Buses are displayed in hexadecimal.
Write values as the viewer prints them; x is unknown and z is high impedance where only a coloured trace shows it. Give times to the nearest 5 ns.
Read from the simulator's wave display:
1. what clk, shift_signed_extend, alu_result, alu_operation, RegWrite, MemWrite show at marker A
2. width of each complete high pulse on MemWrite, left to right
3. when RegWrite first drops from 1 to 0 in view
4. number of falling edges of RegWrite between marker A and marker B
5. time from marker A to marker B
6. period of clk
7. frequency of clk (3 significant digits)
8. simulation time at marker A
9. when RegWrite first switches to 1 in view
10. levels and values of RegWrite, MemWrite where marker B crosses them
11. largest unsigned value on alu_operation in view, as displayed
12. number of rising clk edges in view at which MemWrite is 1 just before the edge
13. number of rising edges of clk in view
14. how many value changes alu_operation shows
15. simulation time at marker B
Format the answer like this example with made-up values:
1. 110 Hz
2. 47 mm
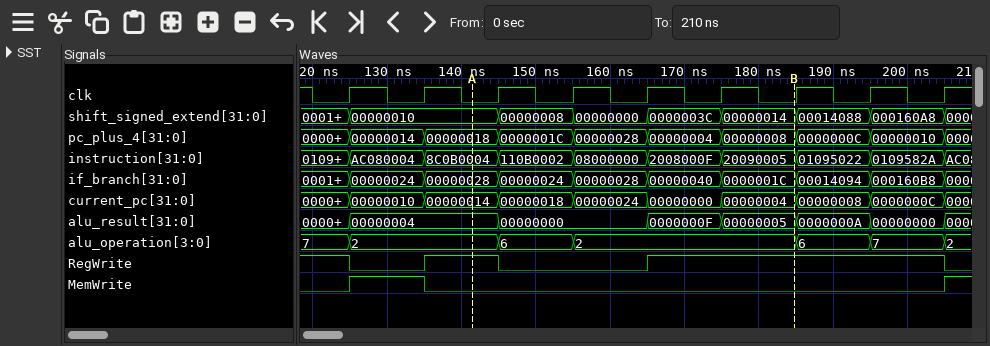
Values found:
1. clk=0, shift_signed_extend=00000010, alu_result=00000004, alu_operation=2, RegWrite=1, MemWrite=0
2. 10 ns
3. 125 ns
4. 1
5. 45 ns
6. 10 ns
7. 100 MHz
8. 140 ns
9. 135 ns
10. RegWrite=1, MemWrite=0
11. 7
12. 1
13. 9
14. 6
15. 185 ns
